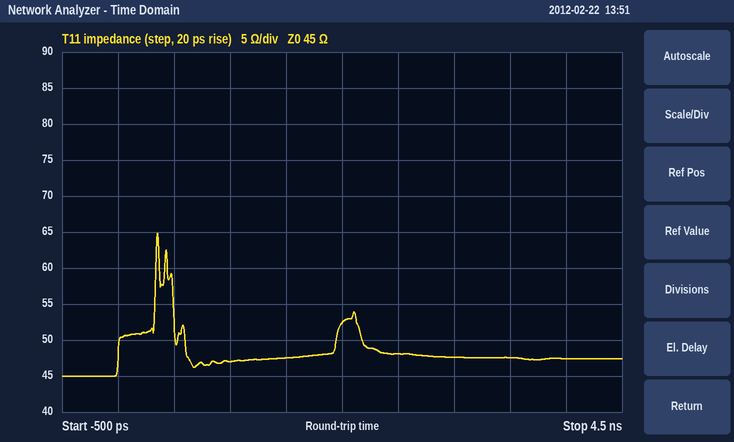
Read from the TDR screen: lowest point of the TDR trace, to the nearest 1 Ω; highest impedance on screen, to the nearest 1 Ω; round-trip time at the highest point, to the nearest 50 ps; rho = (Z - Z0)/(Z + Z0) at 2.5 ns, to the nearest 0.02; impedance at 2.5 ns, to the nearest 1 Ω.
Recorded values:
45 Ω
65 Ω
350 ps
+0.04
48 Ω
